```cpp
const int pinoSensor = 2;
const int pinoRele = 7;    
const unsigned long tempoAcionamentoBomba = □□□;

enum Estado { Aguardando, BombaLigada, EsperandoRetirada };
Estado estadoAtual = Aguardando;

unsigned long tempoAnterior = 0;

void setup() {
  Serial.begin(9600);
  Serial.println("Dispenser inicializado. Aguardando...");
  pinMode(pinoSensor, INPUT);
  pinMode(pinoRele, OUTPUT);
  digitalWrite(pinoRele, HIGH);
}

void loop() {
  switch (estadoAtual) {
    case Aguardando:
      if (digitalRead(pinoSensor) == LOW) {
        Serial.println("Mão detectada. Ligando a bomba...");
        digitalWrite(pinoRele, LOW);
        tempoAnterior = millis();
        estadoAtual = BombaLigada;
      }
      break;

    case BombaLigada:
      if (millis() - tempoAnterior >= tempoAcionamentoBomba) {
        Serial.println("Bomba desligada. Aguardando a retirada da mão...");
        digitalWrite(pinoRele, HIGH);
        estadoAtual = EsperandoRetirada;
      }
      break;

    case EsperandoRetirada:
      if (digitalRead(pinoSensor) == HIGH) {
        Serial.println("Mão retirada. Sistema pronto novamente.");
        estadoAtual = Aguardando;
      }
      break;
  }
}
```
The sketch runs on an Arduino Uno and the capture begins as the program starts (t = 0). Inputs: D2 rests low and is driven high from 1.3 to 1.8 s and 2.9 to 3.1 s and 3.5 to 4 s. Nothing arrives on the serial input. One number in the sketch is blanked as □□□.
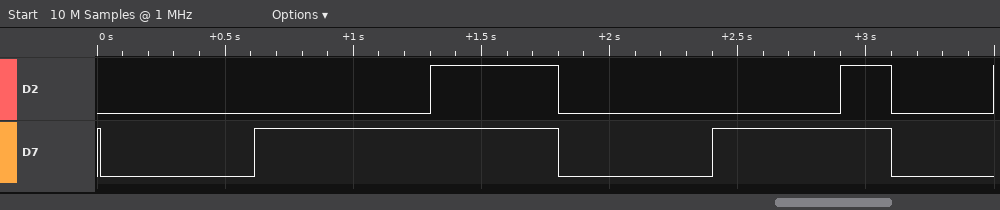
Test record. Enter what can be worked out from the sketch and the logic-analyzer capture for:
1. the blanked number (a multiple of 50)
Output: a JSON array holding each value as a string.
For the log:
["600"]
